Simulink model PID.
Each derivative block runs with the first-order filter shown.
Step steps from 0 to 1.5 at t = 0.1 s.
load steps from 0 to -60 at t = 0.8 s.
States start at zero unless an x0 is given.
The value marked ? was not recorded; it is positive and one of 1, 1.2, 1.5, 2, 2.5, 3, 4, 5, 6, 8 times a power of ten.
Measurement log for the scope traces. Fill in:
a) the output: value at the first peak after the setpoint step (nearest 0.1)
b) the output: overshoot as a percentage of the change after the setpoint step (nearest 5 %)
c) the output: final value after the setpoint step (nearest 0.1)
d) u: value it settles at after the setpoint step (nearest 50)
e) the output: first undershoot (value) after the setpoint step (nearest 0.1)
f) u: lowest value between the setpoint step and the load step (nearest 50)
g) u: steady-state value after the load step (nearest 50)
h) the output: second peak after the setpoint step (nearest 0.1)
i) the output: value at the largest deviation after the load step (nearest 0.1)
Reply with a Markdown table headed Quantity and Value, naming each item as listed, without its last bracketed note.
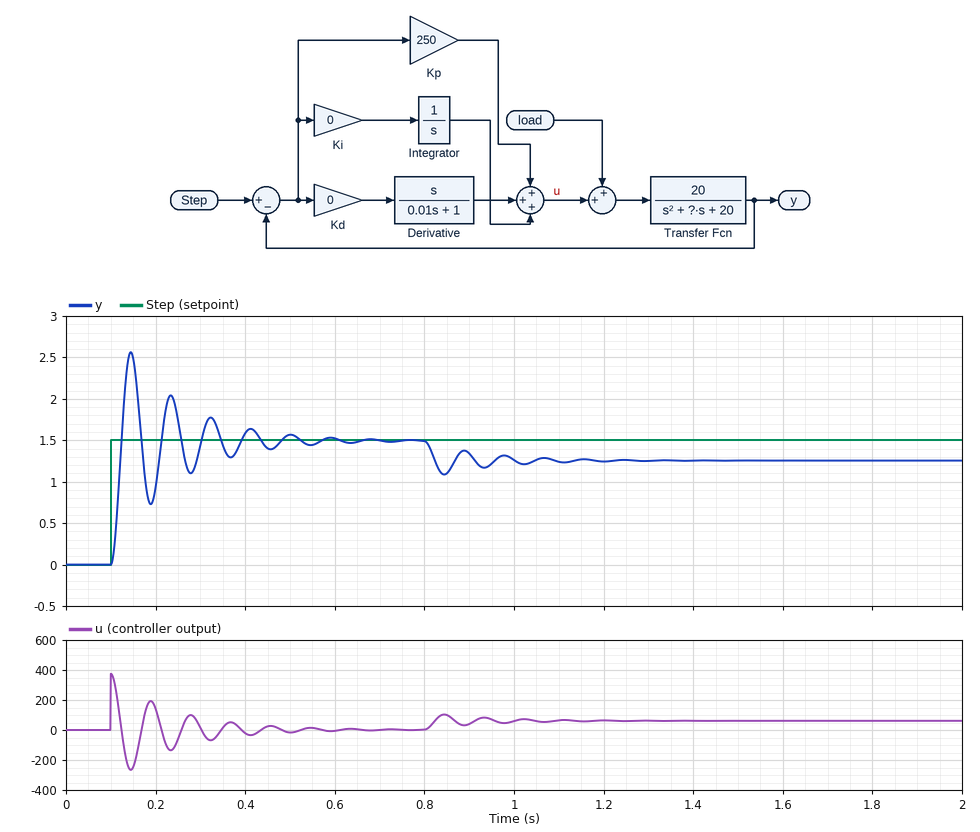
| Quantity | Value |
|---|---|
| the output: value at the first peak after the setpoint step | 2.6 |
| the output: overshoot as a percentage of the change after the setpoint step | 70 % |
| the output: final value after the setpoint step | 1.5 |
| u: value it settles at after the setpoint step | 0 |
| the output: first undershoot (value) after the setpoint step | 0.7 |
| u: lowest value between the setpoint step and the load step | -250 |
| u: steady-state value after the load step | 50 |
| the output: second peak after the setpoint step | 2.0 |
| the output: value at the largest deviation after the load step | 1.1 |
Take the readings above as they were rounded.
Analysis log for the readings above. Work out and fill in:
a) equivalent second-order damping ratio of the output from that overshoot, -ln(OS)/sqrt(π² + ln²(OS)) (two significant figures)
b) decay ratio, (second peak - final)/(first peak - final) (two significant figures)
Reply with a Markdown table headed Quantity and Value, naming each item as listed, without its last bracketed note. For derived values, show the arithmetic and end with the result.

| Quantity | Value |
|---|---|
| equivalent second-order damping ratio of the output from that overshoot, -ln(OS)/sqrt(π² + ln²(OS)) | ln(0.7) = -0.357; 0.357 / sqrt(9.870 + 0.127) = 0.11 |
| decay ratio, (second peak - final)/(first peak - final) | (2 - 1.5) / (2.6 - 1.5) = 0.45 |
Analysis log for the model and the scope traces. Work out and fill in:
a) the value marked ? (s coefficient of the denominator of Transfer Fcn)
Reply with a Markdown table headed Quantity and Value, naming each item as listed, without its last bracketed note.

| Quantity | Value |
|---|---|
| the value marked ? | 15 |
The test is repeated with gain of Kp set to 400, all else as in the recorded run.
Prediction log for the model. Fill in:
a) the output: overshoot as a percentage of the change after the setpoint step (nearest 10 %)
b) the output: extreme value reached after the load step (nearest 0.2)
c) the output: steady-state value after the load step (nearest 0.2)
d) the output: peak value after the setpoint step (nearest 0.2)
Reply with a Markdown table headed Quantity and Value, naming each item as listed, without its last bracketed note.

| Quantity | Value |
|---|---|
| the output: overshoot as a percentage of the change after the setpoint step | 80 % |
| the output: extreme value reached after the load step | 1.2 |
| the output: steady-state value after the load step | 1.4 |
| the output: peak value after the setpoint step | 2.6 |
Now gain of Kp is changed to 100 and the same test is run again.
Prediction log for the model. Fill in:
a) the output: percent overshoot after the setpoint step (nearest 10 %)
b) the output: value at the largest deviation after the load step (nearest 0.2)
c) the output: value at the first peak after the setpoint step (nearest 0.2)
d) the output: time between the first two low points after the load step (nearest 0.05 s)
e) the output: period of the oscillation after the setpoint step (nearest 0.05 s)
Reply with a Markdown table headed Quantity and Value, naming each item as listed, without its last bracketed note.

| Quantity | Value |
|---|---|
| the output: percent overshoot after the setpoint step | 60 % |
| the output: value at the largest deviation after the load step | 0.6 |
| the output: value at the first peak after the setpoint step | 2.4 |
| the output: time between the first two low points after the load step | 0.15 s |
| the output: period of the oscillation after the setpoint step | 0.15 s |
